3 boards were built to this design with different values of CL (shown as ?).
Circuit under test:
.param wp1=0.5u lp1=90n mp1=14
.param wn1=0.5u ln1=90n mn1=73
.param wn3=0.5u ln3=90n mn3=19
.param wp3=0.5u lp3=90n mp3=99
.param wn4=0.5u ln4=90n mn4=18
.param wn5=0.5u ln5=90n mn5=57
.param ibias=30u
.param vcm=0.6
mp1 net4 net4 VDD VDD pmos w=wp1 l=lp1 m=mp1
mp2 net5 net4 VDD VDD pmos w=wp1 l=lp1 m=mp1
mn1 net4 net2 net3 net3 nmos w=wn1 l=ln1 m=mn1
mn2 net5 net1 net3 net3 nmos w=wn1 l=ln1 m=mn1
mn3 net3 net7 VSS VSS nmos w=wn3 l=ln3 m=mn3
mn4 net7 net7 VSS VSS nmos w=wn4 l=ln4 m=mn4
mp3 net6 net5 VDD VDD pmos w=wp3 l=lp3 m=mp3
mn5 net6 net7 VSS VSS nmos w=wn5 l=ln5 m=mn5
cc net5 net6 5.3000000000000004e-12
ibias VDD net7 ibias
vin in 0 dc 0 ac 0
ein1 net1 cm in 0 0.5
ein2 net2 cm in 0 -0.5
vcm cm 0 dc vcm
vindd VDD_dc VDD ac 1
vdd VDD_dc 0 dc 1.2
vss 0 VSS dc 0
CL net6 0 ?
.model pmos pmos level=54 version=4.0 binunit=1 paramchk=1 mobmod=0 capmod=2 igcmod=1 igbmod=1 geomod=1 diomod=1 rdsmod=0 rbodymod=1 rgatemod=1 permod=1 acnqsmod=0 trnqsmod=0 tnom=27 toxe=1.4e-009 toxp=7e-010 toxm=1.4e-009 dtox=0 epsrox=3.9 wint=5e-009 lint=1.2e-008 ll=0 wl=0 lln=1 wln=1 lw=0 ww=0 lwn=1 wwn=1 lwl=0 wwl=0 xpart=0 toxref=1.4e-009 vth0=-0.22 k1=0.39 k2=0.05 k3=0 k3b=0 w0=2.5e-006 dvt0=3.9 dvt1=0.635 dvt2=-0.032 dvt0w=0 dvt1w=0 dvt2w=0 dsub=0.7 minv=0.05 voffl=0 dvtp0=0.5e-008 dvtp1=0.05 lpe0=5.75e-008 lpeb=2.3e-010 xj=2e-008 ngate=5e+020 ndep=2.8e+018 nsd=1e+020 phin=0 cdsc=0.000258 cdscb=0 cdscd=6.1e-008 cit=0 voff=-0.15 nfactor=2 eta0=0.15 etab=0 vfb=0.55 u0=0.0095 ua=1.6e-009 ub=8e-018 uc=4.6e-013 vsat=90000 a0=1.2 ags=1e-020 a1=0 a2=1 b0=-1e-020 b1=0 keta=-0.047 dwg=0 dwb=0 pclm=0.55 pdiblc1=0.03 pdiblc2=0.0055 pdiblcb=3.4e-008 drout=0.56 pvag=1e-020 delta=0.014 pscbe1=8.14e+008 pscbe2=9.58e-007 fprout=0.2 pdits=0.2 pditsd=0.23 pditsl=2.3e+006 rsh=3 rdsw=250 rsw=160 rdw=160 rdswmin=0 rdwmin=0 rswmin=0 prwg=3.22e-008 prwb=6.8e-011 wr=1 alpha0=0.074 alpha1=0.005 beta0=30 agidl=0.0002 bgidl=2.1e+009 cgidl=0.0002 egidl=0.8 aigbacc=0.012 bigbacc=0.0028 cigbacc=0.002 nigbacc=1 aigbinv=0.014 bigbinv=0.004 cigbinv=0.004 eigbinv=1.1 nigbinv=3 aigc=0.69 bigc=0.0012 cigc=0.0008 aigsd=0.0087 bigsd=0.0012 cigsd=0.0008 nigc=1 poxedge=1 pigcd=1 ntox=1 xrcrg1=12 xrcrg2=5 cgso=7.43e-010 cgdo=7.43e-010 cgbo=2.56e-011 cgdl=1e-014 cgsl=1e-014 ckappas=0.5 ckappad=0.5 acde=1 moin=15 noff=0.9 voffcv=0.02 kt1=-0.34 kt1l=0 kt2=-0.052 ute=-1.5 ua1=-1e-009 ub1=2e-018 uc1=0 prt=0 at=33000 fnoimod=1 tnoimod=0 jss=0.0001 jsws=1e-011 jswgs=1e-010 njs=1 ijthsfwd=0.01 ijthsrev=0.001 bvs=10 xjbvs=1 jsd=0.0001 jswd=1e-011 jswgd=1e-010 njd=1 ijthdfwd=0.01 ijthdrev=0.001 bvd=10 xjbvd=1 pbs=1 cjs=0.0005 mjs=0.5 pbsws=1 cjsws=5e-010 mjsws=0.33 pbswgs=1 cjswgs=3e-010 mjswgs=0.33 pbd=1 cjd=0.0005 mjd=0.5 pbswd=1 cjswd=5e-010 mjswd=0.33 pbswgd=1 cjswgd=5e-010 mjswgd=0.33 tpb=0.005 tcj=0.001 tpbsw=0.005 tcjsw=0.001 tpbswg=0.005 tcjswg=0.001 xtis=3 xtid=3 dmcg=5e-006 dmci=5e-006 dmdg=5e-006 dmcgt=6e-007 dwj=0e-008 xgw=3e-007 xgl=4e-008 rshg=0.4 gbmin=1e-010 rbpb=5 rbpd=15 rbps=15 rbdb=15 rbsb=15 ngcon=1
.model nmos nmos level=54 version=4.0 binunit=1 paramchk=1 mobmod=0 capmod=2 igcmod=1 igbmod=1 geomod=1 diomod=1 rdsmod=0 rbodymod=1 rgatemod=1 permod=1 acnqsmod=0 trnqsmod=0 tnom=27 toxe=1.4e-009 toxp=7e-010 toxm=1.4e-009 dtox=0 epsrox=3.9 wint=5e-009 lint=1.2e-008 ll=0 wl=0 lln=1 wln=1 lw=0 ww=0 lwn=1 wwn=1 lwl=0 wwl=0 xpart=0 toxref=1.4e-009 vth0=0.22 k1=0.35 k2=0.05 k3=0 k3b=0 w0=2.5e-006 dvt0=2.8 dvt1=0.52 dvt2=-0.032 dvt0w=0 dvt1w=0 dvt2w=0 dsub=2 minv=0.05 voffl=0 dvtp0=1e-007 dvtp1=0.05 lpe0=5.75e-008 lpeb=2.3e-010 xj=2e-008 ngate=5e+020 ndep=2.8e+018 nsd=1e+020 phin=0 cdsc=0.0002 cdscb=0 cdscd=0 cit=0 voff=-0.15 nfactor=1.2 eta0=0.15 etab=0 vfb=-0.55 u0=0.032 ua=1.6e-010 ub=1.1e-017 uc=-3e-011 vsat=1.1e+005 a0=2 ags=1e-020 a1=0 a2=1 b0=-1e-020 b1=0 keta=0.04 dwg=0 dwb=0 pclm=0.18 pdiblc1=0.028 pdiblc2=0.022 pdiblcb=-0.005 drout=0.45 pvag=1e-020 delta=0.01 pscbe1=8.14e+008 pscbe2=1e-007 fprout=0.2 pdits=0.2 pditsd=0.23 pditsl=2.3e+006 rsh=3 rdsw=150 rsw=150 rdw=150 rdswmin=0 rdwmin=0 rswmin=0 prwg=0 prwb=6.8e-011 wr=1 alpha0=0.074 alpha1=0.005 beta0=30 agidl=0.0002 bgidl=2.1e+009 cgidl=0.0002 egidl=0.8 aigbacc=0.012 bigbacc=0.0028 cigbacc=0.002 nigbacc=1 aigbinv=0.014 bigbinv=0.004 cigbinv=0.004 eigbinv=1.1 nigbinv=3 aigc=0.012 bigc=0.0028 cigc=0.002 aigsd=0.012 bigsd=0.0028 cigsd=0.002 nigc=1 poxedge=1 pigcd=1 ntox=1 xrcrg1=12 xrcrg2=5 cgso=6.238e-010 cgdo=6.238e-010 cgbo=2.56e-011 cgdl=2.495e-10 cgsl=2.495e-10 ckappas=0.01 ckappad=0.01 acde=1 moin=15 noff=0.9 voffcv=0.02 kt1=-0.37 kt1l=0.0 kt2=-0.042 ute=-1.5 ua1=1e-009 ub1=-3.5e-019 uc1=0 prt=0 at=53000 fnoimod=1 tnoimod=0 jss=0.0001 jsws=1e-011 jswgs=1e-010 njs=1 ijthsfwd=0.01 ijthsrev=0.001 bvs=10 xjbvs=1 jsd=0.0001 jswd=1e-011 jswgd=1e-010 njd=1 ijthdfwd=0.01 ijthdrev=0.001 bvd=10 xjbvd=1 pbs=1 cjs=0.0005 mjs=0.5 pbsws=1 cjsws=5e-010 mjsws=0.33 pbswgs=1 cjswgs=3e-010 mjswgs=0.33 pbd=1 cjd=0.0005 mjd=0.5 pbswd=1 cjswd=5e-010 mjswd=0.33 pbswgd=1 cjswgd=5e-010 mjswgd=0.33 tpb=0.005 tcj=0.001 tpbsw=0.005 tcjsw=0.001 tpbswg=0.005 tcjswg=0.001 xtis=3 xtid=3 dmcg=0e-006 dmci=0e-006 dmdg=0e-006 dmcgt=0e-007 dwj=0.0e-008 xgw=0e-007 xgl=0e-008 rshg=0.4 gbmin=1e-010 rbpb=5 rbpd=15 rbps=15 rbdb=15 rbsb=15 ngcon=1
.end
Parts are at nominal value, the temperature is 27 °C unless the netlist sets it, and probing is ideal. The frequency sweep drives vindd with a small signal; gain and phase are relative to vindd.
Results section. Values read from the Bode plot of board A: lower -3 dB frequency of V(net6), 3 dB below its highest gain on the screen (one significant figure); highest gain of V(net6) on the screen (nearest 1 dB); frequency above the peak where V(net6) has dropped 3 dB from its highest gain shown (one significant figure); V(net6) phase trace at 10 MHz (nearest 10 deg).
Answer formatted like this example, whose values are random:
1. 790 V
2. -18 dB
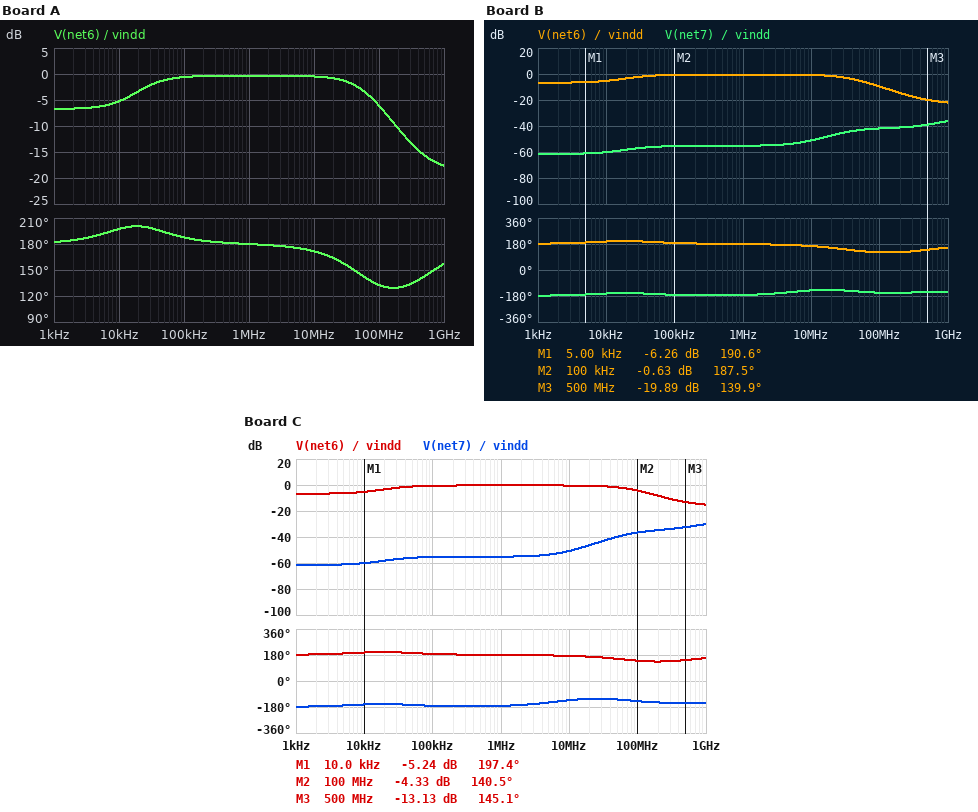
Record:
1. 20 kHz
2. 0 dB
3. 60 MHz
4. 170 deg
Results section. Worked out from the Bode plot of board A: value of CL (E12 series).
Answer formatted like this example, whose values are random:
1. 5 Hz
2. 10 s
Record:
1. 4.7 pF
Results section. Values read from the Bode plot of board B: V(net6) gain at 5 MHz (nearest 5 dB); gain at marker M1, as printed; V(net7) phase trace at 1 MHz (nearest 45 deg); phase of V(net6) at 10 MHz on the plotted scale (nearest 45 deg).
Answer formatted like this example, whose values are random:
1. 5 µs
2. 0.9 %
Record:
1. 0 dB
2. -6.26 dB
3. -180 deg
4. 180 deg
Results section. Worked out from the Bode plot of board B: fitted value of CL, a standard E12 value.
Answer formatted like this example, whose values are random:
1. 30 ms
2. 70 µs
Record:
1. 8.2 pF
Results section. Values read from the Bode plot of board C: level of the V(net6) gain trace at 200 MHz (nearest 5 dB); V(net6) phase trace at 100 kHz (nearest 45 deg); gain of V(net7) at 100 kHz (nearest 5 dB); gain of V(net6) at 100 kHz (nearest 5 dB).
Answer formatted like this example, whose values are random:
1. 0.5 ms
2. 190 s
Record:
1. -10 dB
2. 180 deg
3. -55 dB
4. 0 dB
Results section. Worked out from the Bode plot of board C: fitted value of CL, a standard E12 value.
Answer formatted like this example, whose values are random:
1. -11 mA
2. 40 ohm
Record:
1. 3.3 pF
